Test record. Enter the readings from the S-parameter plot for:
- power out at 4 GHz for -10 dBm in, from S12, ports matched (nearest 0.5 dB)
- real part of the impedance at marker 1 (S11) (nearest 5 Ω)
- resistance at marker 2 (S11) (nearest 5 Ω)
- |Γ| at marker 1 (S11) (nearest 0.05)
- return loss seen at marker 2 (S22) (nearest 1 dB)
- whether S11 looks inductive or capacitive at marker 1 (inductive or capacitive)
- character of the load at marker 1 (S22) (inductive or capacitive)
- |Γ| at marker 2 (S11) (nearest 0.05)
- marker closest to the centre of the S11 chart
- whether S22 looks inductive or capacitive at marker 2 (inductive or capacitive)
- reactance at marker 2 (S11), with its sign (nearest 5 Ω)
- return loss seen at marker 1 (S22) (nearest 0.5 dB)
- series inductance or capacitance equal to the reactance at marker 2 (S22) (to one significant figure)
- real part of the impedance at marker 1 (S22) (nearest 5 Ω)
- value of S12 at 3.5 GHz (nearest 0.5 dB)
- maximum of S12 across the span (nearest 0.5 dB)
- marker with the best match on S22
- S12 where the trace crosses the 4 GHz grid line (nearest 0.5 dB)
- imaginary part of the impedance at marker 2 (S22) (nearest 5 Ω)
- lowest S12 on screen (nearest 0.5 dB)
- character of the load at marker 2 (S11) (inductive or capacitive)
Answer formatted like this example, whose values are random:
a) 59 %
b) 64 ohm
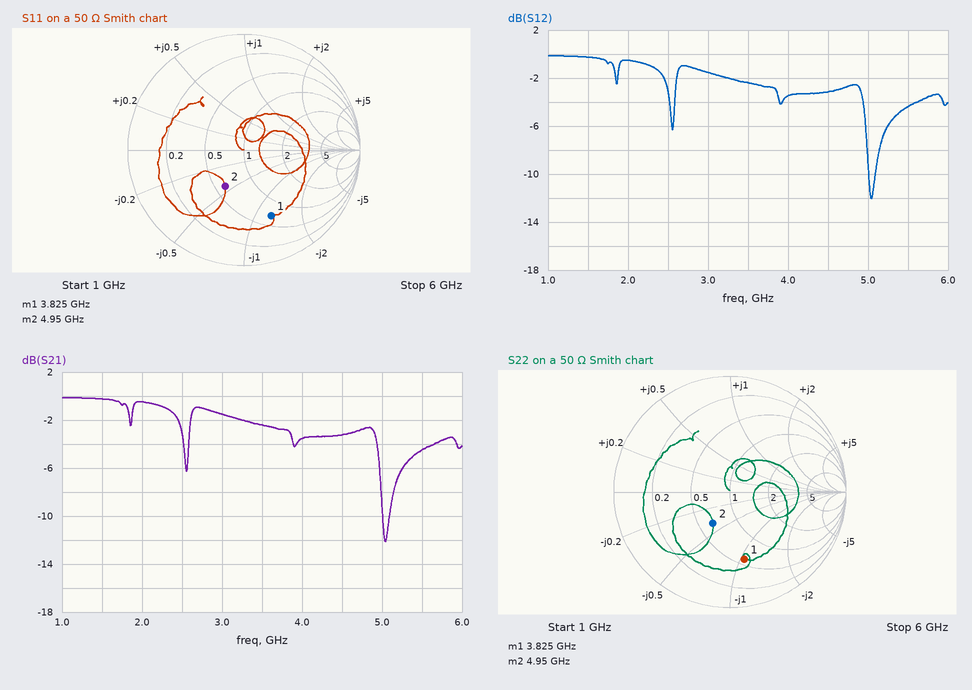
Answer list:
a) -13.5 dBm
b) 35 Ω
c) 30 Ω
d) 0.60
e) 10 dB
f) capacitive
g) capacitive
h) 0.35
i) marker 2
j) capacitive
k) -20 Ω
l) 4.5 dB
m) 2 pF
n) 30 Ω
o) -2.5 dB
p) 0.0 dB
q) marker 2
r) -3.5 dB
s) -20 Ω
t) -12.0 dB
u) capacitive
